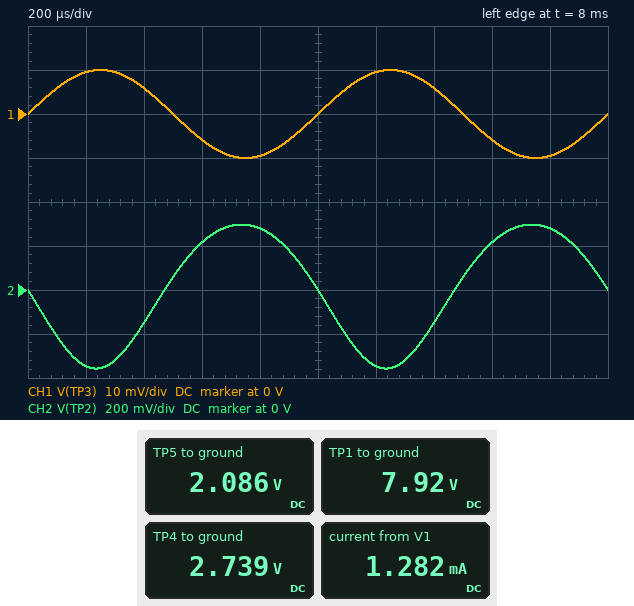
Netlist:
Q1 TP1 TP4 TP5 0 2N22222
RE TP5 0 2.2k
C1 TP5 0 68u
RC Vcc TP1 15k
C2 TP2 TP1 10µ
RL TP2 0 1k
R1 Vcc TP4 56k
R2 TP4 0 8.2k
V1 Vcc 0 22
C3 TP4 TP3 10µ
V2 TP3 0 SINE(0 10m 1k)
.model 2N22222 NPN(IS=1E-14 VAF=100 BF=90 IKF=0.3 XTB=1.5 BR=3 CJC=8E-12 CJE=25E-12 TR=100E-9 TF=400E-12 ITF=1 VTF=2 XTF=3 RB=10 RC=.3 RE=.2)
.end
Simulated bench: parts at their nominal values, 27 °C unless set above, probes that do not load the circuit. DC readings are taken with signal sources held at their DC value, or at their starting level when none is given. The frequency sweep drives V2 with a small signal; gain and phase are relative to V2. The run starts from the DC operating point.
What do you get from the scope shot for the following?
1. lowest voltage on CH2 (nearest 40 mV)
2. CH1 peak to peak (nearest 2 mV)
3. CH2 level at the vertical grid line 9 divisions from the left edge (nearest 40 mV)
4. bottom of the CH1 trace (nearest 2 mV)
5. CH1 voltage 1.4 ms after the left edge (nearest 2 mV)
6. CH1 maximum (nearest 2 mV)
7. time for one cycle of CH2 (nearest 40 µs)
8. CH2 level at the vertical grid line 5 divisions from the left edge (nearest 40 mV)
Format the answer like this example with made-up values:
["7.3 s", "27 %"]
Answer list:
["-360 mV", "20 mV", "280 mV", "-10 mV", "6 mV", "10 mV", "1.00 ms", "0 V"]
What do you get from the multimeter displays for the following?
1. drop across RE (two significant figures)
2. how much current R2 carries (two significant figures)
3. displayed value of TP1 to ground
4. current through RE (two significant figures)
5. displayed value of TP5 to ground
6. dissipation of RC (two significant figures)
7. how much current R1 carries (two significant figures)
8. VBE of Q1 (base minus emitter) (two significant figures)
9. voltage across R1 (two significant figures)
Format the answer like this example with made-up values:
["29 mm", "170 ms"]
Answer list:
["2.1 V", "330 µA", "7.92 V", "950 µA", "2.086 V", "13 mW", "340 µA", "650 mV", "19 V"]
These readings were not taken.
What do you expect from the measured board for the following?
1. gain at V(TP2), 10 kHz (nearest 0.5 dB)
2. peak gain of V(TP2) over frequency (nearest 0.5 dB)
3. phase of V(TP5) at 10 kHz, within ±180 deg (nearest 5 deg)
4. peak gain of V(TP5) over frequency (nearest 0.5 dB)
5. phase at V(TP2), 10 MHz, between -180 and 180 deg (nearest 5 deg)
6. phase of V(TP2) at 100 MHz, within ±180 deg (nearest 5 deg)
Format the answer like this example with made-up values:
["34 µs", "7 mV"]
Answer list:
["30.5 dB", "30.5 dB", "-90 deg", "-1.0 dB", "160 deg", "90 deg"]
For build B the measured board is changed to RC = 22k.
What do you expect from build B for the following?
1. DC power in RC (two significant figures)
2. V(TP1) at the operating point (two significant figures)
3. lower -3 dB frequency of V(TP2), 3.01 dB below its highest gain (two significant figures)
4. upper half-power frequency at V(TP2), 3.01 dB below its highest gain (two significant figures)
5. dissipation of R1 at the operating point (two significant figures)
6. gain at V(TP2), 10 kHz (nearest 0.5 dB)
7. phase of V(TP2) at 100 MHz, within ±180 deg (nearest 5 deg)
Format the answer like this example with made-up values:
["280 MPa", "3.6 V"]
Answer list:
["18 mW", "2.1 V", "130 Hz", "2.7 MHz", "6.7 mW", "23.5 dB", "15 deg"]
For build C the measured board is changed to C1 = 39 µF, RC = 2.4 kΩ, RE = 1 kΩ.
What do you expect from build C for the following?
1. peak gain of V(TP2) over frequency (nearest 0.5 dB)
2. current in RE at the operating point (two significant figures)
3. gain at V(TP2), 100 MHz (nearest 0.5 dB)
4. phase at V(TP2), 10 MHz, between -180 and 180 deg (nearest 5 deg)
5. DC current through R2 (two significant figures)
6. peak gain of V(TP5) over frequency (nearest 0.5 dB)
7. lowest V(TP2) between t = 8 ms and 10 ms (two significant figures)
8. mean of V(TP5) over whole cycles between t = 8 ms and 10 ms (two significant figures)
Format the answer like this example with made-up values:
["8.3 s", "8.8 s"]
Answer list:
["34.5 dB", "2.0 mA", "25.5 dB", "165 deg", "330 µA", "-0.5 dB", "-530 mV", "2.0 V"]
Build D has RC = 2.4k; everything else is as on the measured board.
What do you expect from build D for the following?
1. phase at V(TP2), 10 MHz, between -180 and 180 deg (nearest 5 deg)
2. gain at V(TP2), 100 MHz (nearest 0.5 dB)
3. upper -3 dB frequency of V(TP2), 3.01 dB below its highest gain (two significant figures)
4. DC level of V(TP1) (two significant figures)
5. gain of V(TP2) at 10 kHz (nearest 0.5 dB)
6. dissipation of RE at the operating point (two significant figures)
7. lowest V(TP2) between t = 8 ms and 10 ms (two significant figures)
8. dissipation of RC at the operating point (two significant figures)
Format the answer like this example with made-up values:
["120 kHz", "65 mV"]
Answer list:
["170 deg", "21.5 dB", "54 MHz", "20 V", "28.0 dB", "2.0 mW", "-270 mV", "2.1 mW"]
